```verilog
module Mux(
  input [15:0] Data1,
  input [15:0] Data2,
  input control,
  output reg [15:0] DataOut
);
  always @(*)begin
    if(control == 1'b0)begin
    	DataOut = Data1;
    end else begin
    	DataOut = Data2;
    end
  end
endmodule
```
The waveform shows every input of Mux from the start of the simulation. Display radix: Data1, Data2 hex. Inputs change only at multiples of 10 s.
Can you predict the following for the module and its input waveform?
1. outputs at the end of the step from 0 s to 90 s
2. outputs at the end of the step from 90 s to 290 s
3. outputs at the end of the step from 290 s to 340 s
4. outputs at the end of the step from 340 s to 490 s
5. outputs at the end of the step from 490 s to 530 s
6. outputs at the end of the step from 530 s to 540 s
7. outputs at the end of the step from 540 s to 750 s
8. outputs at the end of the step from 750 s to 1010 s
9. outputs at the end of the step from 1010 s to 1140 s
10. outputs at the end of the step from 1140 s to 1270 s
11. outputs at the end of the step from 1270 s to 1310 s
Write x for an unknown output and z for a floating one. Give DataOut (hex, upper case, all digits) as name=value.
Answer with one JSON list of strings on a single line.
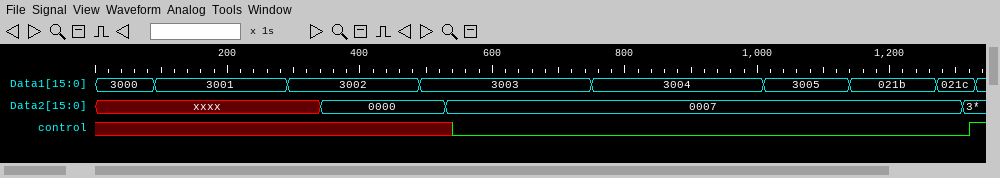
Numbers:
["DataOut=x", "DataOut=x", "DataOut=x", "DataOut=0000", "DataOut=0000", "DataOut=0007", "DataOut=3003", "DataOut=3004", "DataOut=3005", "DataOut=021B", "DataOut=021C"]
